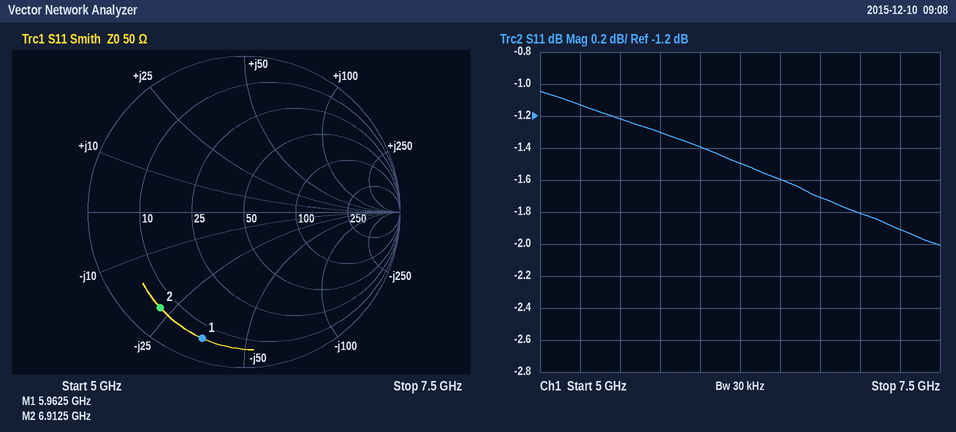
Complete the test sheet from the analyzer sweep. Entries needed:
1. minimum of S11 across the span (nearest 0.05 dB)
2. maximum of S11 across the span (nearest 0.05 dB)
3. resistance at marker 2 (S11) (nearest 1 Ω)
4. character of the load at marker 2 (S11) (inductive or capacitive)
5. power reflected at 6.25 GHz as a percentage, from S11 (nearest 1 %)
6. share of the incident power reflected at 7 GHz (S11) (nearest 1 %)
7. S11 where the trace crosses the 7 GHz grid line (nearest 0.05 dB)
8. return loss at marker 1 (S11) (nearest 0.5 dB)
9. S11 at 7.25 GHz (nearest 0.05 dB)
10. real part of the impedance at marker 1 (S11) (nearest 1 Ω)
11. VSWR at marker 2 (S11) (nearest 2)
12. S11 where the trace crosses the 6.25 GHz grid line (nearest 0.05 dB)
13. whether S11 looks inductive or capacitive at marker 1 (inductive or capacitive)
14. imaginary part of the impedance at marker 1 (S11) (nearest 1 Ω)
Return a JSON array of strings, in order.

["-2.00 dB", "-1.05 dB", "6 Ω", "capacitive", "71 %", "66 %", "-1.80 dB", "1.5 dB", "-1.90 dB", "6 Ω", "10", "-1.50 dB", "capacitive", "-36 Ω"]
